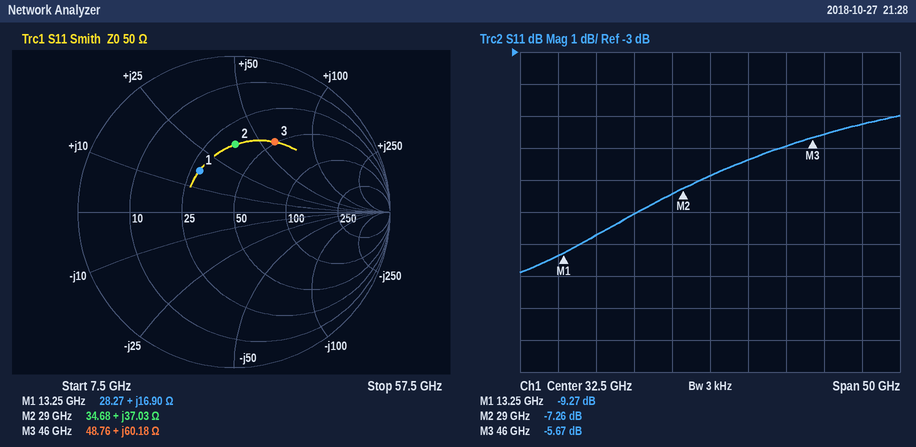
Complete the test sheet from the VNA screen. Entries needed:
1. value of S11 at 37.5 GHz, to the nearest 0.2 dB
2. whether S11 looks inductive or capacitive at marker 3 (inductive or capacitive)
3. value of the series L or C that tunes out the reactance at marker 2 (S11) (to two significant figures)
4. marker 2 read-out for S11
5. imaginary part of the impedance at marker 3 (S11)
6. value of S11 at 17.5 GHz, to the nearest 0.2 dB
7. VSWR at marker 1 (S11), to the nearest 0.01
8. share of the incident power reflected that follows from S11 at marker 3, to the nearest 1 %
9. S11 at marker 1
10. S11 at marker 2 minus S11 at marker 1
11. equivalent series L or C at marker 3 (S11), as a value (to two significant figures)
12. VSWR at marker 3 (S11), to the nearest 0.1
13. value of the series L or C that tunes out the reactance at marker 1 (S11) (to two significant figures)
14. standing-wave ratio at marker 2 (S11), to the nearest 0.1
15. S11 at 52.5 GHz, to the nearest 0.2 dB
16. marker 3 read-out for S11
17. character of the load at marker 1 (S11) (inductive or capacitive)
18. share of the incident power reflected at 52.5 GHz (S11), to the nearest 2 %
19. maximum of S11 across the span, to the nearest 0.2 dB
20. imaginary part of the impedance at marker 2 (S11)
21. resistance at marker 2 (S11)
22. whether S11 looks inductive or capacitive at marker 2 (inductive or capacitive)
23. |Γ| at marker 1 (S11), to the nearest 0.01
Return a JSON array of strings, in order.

["-6.4 dB", "inductive", "150 fF", "-7.26 dB", "+60.18 Ω", "-8.8 dB", "2.05", "27 %", "-9.27 dB", "2.01 dB", "210 pH", "3.2", "710 fF", "2.5", "-5.2 dB", "-5.67 dB", "inductive", "30 %", "-5.0 dB", "+37.03 Ω", "34.68 Ω", "inductive", "0.34"]
